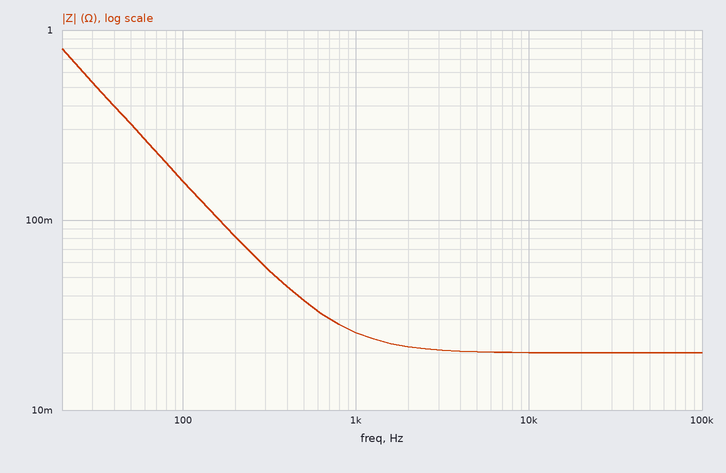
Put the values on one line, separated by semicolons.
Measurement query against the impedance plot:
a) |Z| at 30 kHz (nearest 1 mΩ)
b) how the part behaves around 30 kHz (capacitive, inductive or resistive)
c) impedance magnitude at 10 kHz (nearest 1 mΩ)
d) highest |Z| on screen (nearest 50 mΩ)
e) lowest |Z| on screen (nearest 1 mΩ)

20 mΩ; resistive; 20 mΩ; 800 mΩ; 20 mΩ
